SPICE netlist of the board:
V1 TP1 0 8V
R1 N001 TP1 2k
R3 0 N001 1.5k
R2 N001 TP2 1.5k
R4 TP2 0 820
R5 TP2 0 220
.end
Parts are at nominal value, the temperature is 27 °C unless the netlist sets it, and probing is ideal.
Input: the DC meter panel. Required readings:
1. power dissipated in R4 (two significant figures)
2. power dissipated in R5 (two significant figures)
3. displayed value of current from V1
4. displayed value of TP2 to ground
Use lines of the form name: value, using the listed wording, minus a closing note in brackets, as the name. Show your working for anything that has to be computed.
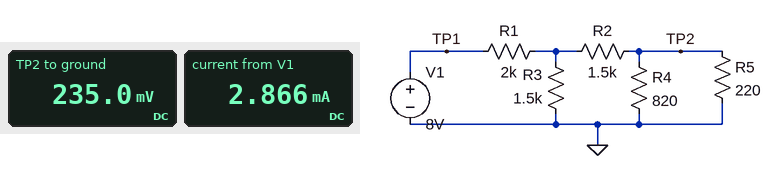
power dissipated in R4: (235 mV)^2 / 820 Ω = 67 µW
power dissipated in R5: (235 mV)^2 / 220 Ω = 250 µW
displayed value of current from V1: 2.866 mA
displayed value of TP2 to ground: 235.0 mV
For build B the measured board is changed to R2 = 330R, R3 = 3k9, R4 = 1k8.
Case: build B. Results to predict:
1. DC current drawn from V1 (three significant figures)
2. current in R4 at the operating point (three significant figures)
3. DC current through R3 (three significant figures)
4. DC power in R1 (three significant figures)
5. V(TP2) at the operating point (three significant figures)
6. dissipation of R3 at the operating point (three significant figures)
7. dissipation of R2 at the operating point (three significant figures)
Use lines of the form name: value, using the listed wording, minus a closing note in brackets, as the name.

DC current drawn from V1: 3.25 mA
current in R4 at the operating point: 312 µA
DC current through R3: 386 µA
DC power in R1: 21.1 mW
V(TP2) at the operating point: 561 mV
dissipation of R3 at the operating point: 581 µW
dissipation of R2 at the operating point: 2.70 mW
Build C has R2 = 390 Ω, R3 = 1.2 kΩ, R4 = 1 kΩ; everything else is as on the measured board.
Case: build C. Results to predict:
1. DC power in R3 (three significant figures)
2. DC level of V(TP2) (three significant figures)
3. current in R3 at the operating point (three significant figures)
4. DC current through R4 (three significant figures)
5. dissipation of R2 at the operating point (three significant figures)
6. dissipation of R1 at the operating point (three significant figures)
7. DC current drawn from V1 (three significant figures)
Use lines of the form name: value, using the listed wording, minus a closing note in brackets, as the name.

DC power in R3: 1.40 mW
DC level of V(TP2): 410 mV
current in R3 at the operating point: 1.08 mA
DC current through R4: 410 µA
dissipation of R2 at the operating point: 2.01 mW
dissipation of R1 at the operating point: 22.5 mW
DC current drawn from V1: 3.35 mA
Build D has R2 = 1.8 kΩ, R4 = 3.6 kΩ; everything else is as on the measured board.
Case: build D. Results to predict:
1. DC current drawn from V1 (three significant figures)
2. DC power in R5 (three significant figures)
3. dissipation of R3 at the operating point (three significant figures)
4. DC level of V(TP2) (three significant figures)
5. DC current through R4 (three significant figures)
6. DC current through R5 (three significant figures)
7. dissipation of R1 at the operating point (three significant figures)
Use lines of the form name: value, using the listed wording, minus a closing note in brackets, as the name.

DC current drawn from V1: 2.80 mA
DC power in R5: 280 µW
dissipation of R3 at the operating point: 3.85 mW
DC level of V(TP2): 248 mV
DC current through R4: 68.9 µA
DC current through R5: 1.13 mA
dissipation of R1 at the operating point: 15.7 mW
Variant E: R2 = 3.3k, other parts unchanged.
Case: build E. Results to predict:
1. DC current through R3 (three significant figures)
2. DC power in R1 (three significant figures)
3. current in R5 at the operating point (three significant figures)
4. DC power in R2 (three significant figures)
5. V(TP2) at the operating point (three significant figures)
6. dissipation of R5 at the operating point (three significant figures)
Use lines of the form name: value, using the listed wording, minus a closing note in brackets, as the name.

DC current through R3: 1.83 mA
DC power in R1: 13.8 mW
current in R5 at the operating point: 624 µA
DC power in R2: 2.07 mW
V(TP2) at the operating point: 137 mV
dissipation of R5 at the operating point: 85.7 µW
